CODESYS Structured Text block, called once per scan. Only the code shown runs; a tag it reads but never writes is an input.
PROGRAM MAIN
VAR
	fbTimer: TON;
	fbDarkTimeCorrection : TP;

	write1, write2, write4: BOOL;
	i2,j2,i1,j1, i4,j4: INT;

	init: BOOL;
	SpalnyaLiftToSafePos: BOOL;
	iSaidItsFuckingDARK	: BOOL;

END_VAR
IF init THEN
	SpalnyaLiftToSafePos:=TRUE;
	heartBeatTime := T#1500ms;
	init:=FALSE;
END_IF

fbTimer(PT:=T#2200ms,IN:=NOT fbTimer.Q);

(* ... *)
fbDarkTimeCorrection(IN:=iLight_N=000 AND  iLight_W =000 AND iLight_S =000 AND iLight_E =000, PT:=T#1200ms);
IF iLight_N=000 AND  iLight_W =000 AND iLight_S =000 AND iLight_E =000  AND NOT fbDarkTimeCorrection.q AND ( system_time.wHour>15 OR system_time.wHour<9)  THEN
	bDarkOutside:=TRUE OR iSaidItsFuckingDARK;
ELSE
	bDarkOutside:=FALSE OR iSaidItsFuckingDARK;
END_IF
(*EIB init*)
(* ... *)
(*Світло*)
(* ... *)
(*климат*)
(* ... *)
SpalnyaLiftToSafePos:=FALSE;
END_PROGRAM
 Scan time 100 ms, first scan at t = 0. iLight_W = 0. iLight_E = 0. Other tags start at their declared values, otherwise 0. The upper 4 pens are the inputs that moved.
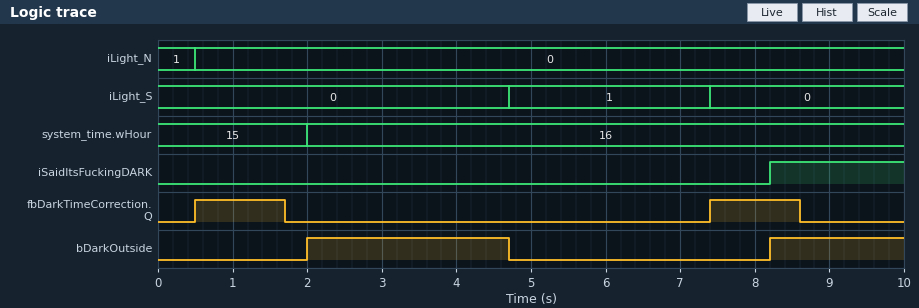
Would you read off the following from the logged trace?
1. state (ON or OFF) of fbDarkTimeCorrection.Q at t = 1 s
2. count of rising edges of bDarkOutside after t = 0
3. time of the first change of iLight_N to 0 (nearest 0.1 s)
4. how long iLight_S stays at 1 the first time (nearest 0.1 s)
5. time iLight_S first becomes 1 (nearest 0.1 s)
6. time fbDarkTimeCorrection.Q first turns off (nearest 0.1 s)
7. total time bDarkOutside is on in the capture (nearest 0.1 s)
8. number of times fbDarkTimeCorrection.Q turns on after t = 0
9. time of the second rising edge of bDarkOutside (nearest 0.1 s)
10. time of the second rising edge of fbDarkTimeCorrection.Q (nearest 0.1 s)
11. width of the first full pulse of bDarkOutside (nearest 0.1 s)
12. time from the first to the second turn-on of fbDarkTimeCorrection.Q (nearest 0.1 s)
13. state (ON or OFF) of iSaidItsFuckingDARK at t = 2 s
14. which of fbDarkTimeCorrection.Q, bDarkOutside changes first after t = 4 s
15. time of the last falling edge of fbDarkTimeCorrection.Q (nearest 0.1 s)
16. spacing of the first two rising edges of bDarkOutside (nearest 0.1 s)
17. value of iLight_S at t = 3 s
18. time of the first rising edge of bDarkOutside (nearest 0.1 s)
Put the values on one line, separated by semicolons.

ON; 2; 0.5 s; 2.7 s; 4.7 s; 1.7 s; 4.5 s; 2; 8.2 s; 7.4 s; 2.7 s; 6.9 s; OFF; bDarkOutside; 8.6 s; 6.2 s; 0; 2.0 s
